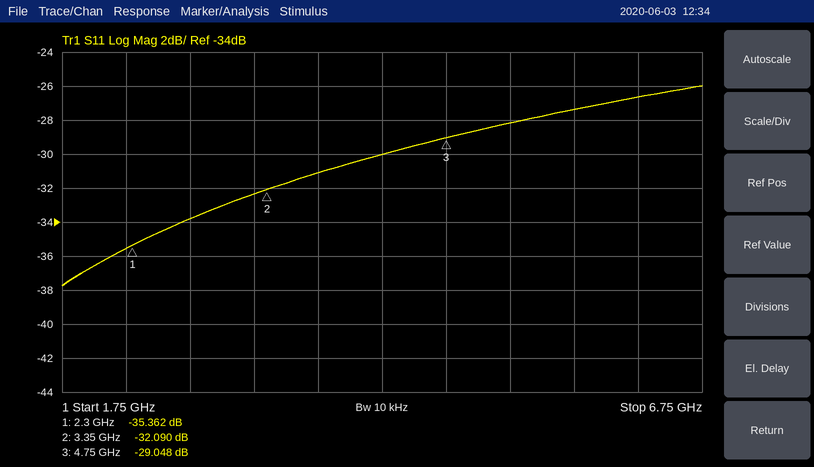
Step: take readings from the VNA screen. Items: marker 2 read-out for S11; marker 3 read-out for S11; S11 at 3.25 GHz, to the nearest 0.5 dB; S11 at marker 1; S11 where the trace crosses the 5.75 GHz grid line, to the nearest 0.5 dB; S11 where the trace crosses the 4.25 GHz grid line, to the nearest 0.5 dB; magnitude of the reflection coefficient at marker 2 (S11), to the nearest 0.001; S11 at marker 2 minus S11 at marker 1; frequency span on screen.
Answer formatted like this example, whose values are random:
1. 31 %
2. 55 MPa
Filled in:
1. -32.090 dB
2. -29.048 dB
3. -32.5 dB
4. -35.362 dB
5. -27.5 dB
6. -30.0 dB
7. 0.025
8. 3.272 dB
9. 5 GHz
